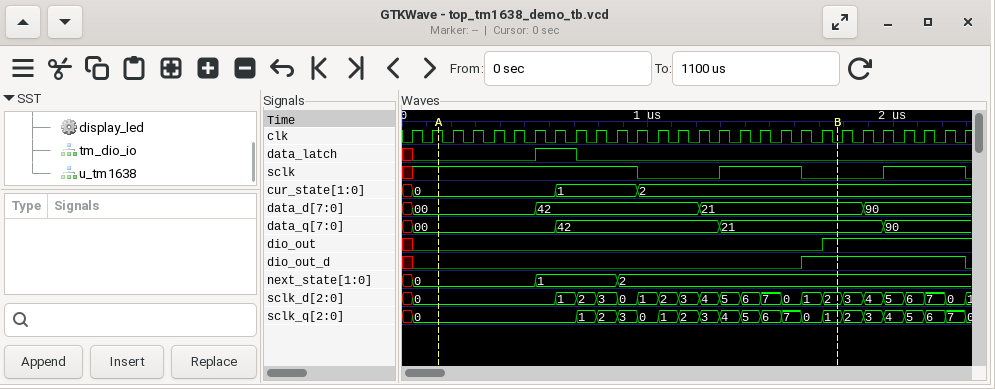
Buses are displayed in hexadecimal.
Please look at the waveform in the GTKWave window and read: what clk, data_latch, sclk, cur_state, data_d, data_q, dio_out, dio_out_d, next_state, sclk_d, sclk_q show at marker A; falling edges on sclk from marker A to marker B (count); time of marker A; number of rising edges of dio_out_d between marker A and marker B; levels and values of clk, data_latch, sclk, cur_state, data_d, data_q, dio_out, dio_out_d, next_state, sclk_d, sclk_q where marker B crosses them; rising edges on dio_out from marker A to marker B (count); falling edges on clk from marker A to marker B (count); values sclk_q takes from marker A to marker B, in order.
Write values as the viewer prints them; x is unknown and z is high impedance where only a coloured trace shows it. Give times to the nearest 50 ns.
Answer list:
clk=1, data_latch=0, sclk=1, cur_state=0, data_d=00, data_q=00, dio_out=0, dio_out_d=0, next_state=0, sclk_d=0, sclk_q=0
2
150 ns
1
clk=0, data_latch=0, sclk=0, cur_state=2, data_d=21, data_q=21, dio_out=1, dio_out_d=1, next_state=2, sclk_d=2, sclk_q=1
1
20
0, 1, 2, 3, 0, 1, 2, 3, 4, 5, 6, 7, 0, 1
